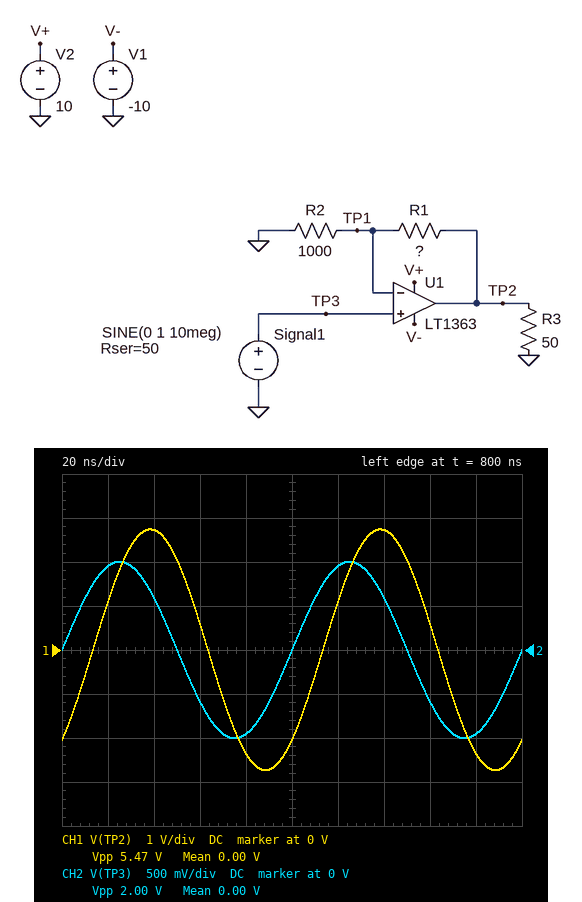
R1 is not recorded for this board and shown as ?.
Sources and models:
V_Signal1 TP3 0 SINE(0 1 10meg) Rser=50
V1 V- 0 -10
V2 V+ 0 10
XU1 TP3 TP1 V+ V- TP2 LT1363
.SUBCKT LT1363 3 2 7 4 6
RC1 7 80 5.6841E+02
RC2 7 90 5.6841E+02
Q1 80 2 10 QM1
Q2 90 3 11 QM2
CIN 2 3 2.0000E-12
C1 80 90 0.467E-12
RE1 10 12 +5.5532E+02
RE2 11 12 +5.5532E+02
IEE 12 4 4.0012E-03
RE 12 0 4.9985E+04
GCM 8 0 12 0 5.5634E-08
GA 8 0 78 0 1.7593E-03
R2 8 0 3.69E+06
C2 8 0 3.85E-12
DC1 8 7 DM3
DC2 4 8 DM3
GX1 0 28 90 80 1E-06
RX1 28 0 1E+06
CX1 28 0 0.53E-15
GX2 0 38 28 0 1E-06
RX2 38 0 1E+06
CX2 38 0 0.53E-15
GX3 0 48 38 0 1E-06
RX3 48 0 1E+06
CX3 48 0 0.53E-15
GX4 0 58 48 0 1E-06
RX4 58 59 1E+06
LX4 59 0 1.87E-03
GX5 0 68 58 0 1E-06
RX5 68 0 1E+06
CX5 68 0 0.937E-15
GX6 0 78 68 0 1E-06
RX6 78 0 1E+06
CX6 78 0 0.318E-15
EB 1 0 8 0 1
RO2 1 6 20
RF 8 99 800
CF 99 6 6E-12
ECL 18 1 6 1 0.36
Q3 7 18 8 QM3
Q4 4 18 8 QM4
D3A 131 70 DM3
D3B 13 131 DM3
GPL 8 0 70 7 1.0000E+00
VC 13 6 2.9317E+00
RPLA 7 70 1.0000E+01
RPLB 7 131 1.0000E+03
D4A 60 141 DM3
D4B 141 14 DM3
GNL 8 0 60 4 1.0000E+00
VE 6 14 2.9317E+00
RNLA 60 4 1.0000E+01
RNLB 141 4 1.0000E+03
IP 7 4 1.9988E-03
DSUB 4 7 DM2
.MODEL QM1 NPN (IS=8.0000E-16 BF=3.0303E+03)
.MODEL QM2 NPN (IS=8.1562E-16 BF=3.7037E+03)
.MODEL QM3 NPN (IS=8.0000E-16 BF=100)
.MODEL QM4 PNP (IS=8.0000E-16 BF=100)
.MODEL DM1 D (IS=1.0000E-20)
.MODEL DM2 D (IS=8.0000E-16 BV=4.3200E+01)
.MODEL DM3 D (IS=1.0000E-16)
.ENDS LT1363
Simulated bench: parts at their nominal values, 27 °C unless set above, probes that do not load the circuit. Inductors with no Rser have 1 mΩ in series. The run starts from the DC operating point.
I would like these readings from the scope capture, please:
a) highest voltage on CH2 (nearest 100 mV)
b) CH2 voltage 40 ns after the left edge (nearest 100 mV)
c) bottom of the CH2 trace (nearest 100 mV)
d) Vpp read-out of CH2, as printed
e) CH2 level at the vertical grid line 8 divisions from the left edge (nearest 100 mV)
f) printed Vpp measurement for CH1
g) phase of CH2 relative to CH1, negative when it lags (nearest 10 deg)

1.0 V
600 mV
-1.0 V
2.00 V
-600 mV
5.47 V
50 deg
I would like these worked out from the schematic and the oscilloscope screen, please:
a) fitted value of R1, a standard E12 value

2.7 kΩ
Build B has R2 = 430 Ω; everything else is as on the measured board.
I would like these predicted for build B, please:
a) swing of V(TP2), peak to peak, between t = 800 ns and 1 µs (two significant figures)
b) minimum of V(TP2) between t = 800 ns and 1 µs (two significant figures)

6.7 V
-3.3 V
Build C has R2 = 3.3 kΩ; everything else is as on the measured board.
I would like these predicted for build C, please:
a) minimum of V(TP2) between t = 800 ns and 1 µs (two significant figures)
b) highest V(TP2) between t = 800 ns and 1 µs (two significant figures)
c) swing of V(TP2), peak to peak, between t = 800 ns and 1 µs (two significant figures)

-1.8 V
1.8 V
3.5 V
